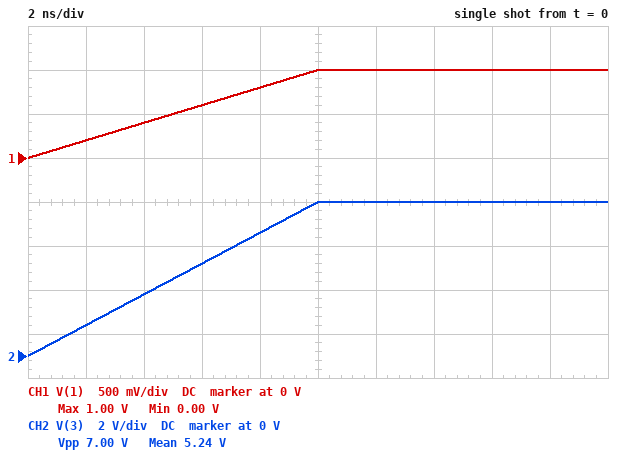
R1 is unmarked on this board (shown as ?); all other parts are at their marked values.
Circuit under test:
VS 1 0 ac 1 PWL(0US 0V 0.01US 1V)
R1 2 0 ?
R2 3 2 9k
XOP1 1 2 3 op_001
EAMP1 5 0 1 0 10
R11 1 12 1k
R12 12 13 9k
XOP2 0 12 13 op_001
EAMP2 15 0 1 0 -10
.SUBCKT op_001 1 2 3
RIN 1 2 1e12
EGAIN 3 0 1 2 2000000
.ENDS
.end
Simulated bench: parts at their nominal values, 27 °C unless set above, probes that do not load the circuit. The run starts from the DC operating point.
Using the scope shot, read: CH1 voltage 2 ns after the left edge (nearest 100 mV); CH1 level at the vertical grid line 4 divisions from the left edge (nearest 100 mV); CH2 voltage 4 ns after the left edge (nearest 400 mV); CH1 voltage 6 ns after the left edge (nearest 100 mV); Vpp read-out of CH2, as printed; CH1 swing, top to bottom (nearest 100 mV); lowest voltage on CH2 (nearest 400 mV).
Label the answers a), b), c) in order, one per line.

a) 200 mV
b) 800 mV
c) 2.8 V
d) 600 mV
e) 7.00 V
f) 1.0 V
g) 0 V
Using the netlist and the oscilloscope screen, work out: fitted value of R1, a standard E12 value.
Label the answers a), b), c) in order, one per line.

a) 1.5 kΩ
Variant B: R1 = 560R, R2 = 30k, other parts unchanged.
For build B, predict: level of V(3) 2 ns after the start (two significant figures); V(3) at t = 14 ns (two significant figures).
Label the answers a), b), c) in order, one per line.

a) 11 V
b) 55 V
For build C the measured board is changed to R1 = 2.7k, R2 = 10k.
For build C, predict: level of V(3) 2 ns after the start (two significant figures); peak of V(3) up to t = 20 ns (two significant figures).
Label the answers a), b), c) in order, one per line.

a) 940 mV
b) 4.7 V
